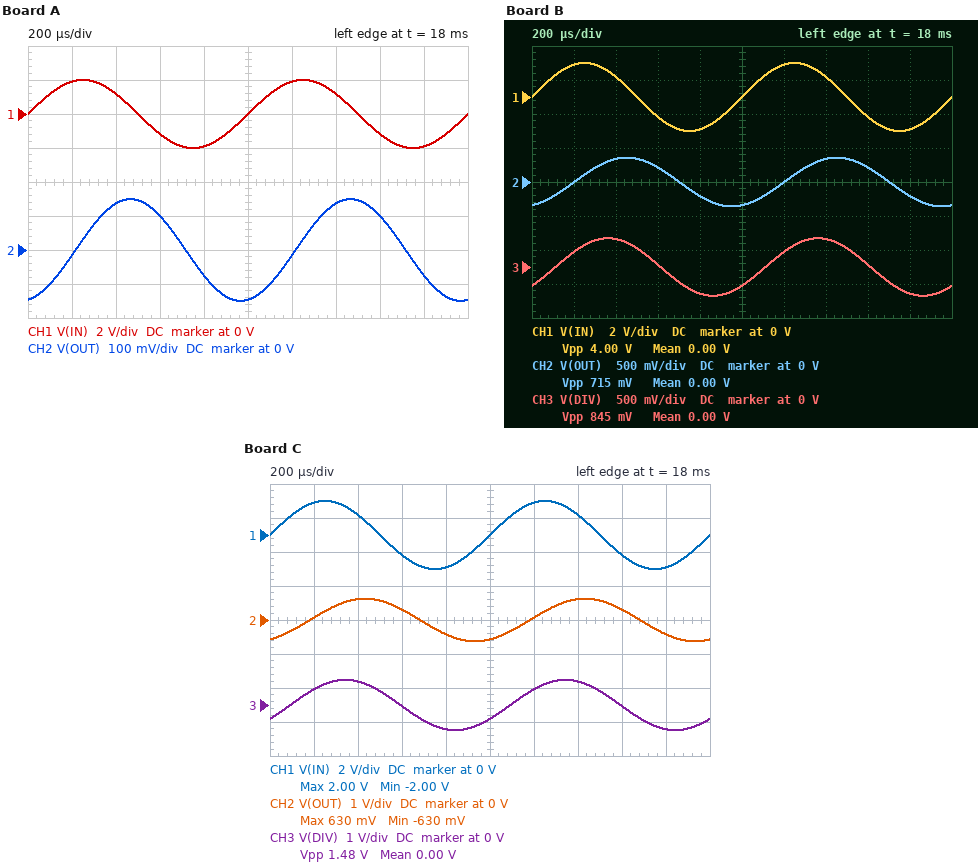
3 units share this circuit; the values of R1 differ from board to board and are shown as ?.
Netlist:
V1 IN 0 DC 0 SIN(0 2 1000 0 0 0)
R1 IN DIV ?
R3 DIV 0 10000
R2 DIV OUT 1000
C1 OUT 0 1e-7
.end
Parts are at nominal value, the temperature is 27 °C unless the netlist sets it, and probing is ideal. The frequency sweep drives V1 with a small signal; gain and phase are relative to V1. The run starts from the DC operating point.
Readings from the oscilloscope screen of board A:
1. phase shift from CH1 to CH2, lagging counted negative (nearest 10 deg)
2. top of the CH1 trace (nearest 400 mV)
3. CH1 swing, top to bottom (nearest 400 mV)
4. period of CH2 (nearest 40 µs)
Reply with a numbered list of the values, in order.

1. -80 deg
2. 2.0 V
3. 4.0 V
4. 1.00 ms
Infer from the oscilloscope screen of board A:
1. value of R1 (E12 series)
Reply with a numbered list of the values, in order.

1. 18 kΩ
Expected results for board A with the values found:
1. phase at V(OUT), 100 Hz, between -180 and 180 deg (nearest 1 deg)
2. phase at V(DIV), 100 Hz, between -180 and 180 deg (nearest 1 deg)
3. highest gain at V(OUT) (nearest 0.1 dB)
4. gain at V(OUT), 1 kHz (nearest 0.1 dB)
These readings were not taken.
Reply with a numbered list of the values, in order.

1. -25 deg
2. -21 deg
3. -8.9 dB
4. -22.5 dB
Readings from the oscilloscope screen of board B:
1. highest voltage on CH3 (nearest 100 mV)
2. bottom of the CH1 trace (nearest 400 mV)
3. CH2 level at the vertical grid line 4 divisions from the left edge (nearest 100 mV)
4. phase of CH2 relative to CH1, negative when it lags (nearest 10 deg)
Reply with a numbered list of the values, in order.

1. 400 mV
2. -2.0 V
3. -200 mV
4. -70 deg
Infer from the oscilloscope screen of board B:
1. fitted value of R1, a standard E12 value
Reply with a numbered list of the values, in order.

1. 6.8 kΩ
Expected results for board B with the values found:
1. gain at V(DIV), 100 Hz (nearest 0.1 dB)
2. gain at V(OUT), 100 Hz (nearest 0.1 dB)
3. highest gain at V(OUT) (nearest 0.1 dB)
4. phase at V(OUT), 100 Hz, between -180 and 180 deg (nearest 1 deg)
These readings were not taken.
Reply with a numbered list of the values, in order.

1. -4.9 dB
2. -4.9 dB
3. -4.5 dB
4. -18 deg
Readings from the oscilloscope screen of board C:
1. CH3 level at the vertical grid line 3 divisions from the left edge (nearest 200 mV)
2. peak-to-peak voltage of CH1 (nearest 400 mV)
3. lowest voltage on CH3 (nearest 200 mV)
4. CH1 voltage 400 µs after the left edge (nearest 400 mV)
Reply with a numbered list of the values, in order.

1. 0 V
2. 4.0 V
3. -800 mV
4. 1.2 V
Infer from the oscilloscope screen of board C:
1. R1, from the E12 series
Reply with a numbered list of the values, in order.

1. 3.3 kΩ
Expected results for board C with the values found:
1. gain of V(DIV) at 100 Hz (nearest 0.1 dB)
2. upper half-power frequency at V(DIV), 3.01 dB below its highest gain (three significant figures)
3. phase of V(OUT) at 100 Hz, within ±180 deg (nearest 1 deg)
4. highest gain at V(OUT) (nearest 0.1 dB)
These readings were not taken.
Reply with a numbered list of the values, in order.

1. -2.7 dB
2. 500 Hz
3. -12 deg
4. -2.5 dB
